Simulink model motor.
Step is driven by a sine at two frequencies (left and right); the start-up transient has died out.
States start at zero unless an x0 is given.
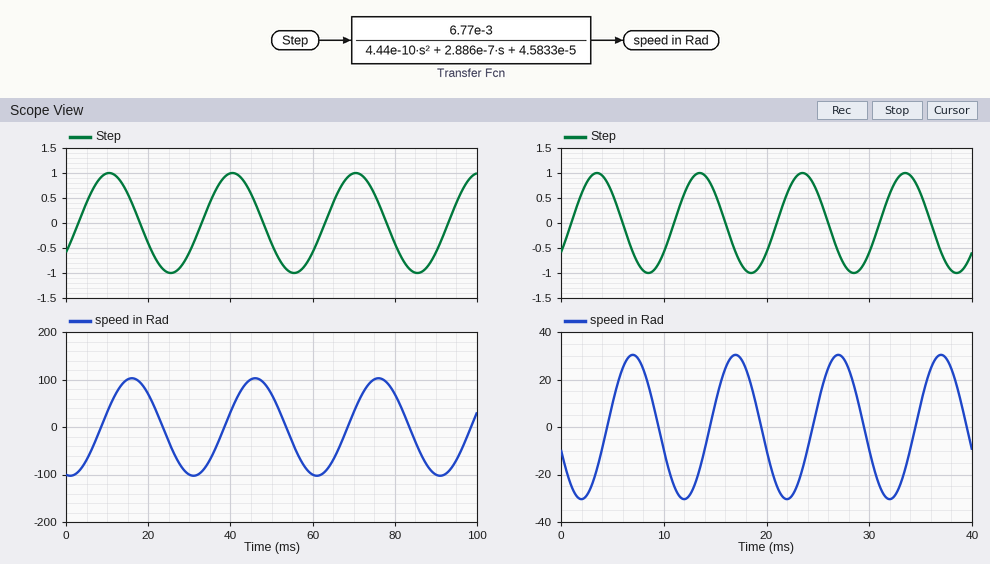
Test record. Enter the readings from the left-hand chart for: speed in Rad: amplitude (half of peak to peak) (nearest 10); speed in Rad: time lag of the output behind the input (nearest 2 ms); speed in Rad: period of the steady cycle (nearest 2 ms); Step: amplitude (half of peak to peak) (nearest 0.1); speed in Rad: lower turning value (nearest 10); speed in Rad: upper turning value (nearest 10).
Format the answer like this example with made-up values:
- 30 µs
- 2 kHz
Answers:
- 100
- 6 ms
- 30 ms
- 1.0
- -100
- 100
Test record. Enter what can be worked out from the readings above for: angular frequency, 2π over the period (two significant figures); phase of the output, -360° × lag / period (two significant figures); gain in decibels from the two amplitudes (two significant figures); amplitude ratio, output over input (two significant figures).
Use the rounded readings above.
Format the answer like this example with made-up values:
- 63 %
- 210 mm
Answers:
- 0.21 rad/ms
- -72°
- 40 dB
- 100
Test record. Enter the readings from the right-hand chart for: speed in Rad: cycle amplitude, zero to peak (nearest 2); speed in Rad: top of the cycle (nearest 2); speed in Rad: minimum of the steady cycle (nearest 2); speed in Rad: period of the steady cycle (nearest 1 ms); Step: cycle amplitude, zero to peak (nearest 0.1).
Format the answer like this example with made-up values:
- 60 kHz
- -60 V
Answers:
- 30
- 30
- -30
- 10 ms
- 1.0
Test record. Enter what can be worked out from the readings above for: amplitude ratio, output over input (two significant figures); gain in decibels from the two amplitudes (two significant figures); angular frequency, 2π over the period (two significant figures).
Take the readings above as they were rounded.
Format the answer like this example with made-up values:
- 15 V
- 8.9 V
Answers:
- 30
- 30 dB
- 0.63 rad/ms
